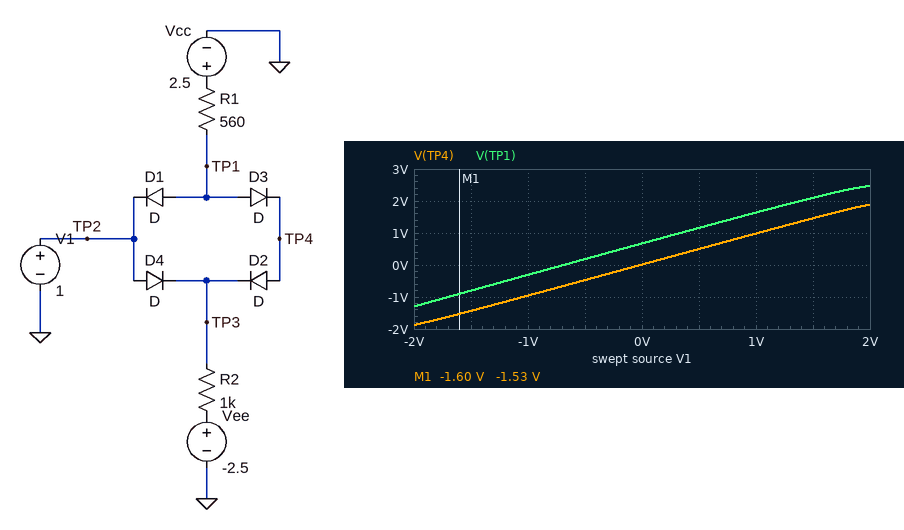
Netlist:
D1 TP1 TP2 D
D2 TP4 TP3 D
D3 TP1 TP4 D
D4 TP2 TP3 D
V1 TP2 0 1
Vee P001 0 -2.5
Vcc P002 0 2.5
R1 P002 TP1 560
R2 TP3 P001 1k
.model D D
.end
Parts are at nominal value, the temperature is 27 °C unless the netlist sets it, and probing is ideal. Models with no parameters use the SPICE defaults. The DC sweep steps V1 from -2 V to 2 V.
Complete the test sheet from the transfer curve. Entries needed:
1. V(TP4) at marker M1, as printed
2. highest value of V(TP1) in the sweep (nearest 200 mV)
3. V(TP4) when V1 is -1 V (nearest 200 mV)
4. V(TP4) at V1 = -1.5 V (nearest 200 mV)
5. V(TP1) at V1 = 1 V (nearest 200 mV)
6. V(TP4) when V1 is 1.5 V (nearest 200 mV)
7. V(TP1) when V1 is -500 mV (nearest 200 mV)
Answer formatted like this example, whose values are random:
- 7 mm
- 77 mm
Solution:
- -1.53 V
- 2.4 V
- -1.0 V
- -1.4 V
- 1.6 V
- 1.4 V
- 200 mV
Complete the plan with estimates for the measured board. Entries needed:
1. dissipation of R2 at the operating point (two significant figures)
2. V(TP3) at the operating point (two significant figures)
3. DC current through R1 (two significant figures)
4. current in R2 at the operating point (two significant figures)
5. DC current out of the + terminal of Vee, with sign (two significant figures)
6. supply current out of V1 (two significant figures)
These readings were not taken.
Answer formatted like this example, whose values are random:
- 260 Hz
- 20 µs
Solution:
- 8.0 mW
- 330 mV
- 1.5 mA
- 2.8 mA
- -2.8 mA
- 1.3 mA
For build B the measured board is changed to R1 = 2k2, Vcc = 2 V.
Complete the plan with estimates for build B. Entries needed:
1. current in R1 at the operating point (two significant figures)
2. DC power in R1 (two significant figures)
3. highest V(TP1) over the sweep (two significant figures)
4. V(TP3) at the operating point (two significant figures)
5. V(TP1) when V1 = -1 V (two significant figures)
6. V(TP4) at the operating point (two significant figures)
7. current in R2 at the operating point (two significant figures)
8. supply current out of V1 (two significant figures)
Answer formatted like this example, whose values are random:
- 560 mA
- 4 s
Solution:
- 210 µA
- 94 µW
- 2.0 V
- 320 mV
- -360 mV
- 930 mV
- 2.8 mA
- 2.6 mA
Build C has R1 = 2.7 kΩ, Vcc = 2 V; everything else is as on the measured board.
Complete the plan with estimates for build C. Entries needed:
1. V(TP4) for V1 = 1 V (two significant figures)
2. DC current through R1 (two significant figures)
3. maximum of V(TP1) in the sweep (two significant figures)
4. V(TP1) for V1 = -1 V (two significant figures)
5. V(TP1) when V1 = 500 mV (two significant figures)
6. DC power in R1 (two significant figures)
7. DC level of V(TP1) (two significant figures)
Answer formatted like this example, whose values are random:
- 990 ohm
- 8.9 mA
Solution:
- 930 mV
- 170 µA
- 2.0 V
- -370 mV
- 1.1 V
- 80 µW
- 1.5 V
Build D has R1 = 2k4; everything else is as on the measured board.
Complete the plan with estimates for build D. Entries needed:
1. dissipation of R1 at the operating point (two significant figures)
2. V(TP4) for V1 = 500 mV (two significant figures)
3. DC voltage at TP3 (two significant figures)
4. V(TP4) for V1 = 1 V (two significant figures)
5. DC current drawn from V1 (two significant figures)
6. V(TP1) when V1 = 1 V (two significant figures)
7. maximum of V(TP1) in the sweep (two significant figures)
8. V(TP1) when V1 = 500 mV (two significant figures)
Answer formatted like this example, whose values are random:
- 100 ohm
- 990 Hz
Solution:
- 360 µW
- 460 mV
- 320 mV
- 950 mV
- 2.4 mA
- 1.6 V
- 2.4 V
- 1.1 V
